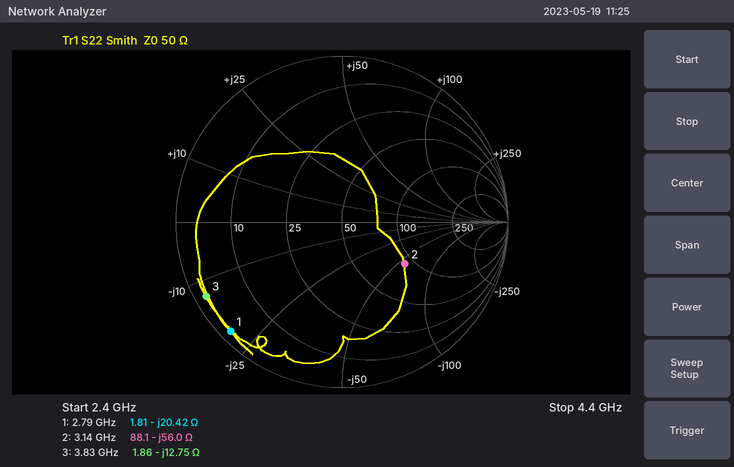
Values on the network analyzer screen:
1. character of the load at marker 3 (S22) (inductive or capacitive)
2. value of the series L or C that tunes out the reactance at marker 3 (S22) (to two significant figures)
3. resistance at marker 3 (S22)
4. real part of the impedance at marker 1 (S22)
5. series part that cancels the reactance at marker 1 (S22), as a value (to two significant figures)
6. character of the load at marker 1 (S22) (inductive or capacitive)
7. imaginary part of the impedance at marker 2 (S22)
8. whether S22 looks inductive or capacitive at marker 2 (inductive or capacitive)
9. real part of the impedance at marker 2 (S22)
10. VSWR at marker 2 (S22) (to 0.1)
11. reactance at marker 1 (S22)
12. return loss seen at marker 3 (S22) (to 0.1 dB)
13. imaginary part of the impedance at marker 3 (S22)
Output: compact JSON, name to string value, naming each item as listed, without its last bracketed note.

{"character of the load at marker 3 (S22)": "capacitive", "value of the series L or C that tunes out the reactance at marker 3 (S22)": "530 pH", "resistance at marker 3": "1.86 Ω", "real part of the impedance at marker 1": "1.81 Ω", "series part that cancels the reactance at marker 1 (S22), as a value": "1.2 nH", "character of the load at marker 1 (S22)": "capacitive", "imaginary part of the impedance at marker 2": "-56.0 Ω", "whether S22 looks inductive or capacitive at marker 2": "capacitive", "real part of the impedance at marker 2": "88.1 Ω", "VSWR at marker 2 (S22)": "2.7", "reactance at marker 1": "-20.42 Ω", "return loss seen at marker 3 (S22)": "0.6 dB", "imaginary part of the impedance at marker 3": "-12.75 Ω"}
